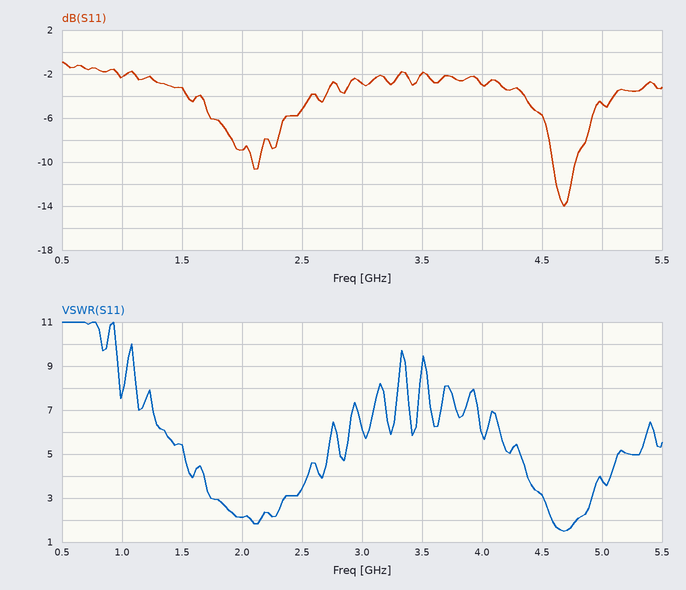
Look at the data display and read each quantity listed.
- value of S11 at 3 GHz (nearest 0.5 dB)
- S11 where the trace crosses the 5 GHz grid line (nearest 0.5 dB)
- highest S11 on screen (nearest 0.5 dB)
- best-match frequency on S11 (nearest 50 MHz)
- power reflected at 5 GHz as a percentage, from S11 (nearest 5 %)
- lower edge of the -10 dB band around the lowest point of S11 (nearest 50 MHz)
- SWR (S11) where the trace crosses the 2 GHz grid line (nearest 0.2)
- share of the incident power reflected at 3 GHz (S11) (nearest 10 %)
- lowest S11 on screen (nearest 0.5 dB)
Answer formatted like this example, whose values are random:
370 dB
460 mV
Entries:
-3.0 dB
-4.5 dB
-1.0 dB
4.70 GHz
35 %
4.60 GHz
2.2
50 %
-14.0 dB
